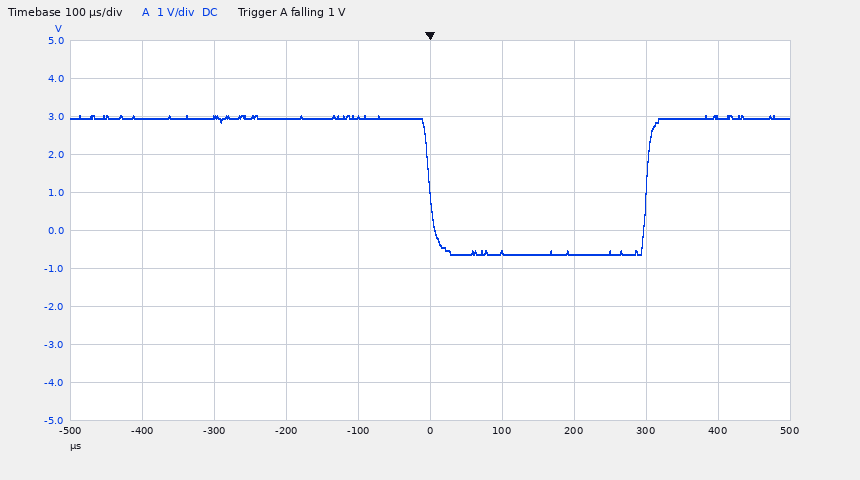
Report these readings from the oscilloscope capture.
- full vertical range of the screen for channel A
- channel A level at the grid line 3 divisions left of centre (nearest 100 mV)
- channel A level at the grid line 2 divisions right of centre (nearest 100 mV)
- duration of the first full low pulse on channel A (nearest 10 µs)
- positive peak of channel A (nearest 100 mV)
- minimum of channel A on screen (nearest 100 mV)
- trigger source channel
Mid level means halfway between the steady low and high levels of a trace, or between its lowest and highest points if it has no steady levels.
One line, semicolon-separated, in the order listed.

10 V; 3.0 V; -600 mV; 300 µs; 3.0 V; -600 mV; channel A
